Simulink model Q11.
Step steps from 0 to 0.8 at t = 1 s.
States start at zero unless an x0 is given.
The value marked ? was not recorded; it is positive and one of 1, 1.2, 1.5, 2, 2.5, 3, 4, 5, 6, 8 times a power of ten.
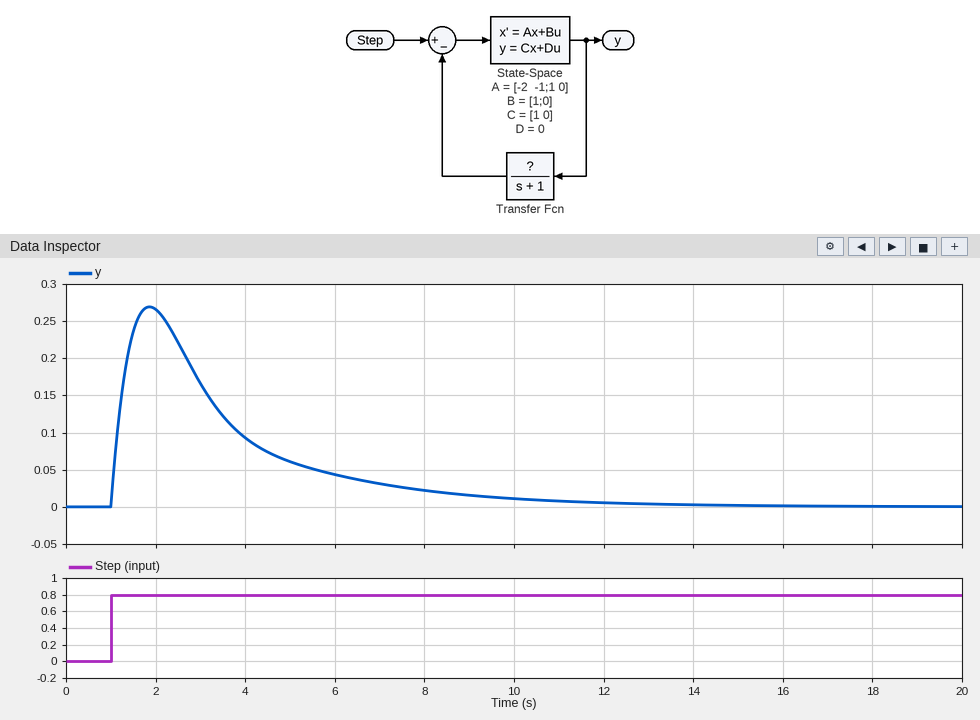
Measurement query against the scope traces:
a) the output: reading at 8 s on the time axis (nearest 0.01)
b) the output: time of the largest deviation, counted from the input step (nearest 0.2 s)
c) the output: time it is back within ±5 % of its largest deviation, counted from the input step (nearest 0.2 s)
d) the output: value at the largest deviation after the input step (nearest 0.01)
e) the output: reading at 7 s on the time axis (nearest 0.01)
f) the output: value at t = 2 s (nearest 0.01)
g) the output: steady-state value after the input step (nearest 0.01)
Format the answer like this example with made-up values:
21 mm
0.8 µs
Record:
0.02
0.8 s
8.4 s
0.27
0.03
0.27
0.00
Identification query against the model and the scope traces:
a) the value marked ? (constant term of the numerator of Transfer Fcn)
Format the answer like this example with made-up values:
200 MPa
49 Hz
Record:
0.8
